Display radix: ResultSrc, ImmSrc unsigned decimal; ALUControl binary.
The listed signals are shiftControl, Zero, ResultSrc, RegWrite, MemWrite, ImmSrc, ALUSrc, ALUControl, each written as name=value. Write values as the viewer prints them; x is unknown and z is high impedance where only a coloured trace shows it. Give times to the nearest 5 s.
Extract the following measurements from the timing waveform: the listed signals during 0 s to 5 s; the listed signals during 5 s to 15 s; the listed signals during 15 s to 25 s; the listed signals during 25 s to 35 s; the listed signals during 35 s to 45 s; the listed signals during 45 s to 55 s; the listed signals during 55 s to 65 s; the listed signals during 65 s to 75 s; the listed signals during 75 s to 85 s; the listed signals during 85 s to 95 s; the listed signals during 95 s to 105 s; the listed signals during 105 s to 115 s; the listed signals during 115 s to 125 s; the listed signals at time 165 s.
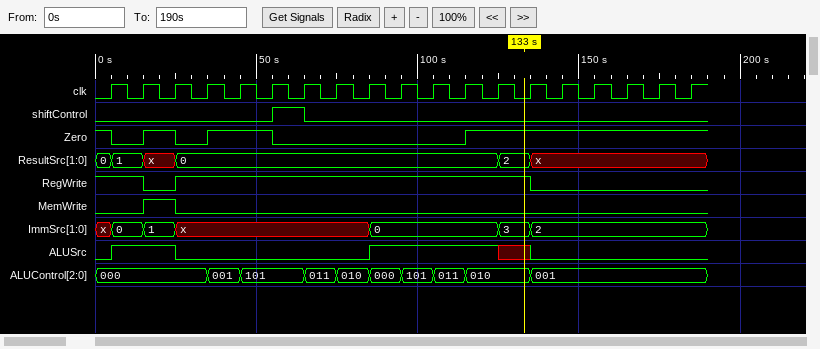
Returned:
shiftControl=0, Zero=1, ResultSrc=0, RegWrite=1, MemWrite=0, ImmSrc=x, ALUSrc=0, ALUControl=000
shiftControl=0, Zero=0, ResultSrc=1, RegWrite=1, MemWrite=0, ImmSrc=0, ALUSrc=1, ALUControl=000
shiftControl=0, Zero=1, ResultSrc=x, RegWrite=0, MemWrite=1, ImmSrc=1, ALUSrc=1, ALUControl=000
shiftControl=0, Zero=0, ResultSrc=0, RegWrite=1, MemWrite=0, ImmSrc=x, ALUSrc=0, ALUControl=000
shiftControl=0, Zero=1, ResultSrc=0, RegWrite=1, MemWrite=0, ImmSrc=x, ALUSrc=0, ALUControl=001
shiftControl=0, Zero=1, ResultSrc=0, RegWrite=1, MemWrite=0, ImmSrc=x, ALUSrc=0, ALUControl=101
shiftControl=1, Zero=0, ResultSrc=0, RegWrite=1, MemWrite=0, ImmSrc=x, ALUSrc=0, ALUControl=101
shiftControl=0, Zero=0, ResultSrc=0, RegWrite=1, MemWrite=0, ImmSrc=x, ALUSrc=0, ALUControl=011
shiftControl=0, Zero=0, ResultSrc=0, RegWrite=1, MemWrite=0, ImmSrc=x, ALUSrc=0, ALUControl=010
shiftControl=0, Zero=0, ResultSrc=0, RegWrite=1, MemWrite=0, ImmSrc=0, ALUSrc=1, ALUControl=000
shiftControl=0, Zero=0, ResultSrc=0, RegWrite=1, MemWrite=0, ImmSrc=0, ALUSrc=1, ALUControl=101
shiftControl=0, Zero=0, ResultSrc=0, RegWrite=1, MemWrite=0, ImmSrc=0, ALUSrc=1, ALUControl=011
shiftControl=0, Zero=1, ResultSrc=0, RegWrite=1, MemWrite=0, ImmSrc=0, ALUSrc=1, ALUControl=010
shiftControl=0, Zero=1, ResultSrc=x, RegWrite=0, MemWrite=0, ImmSrc=2, ALUSrc=0, ALUControl=001
